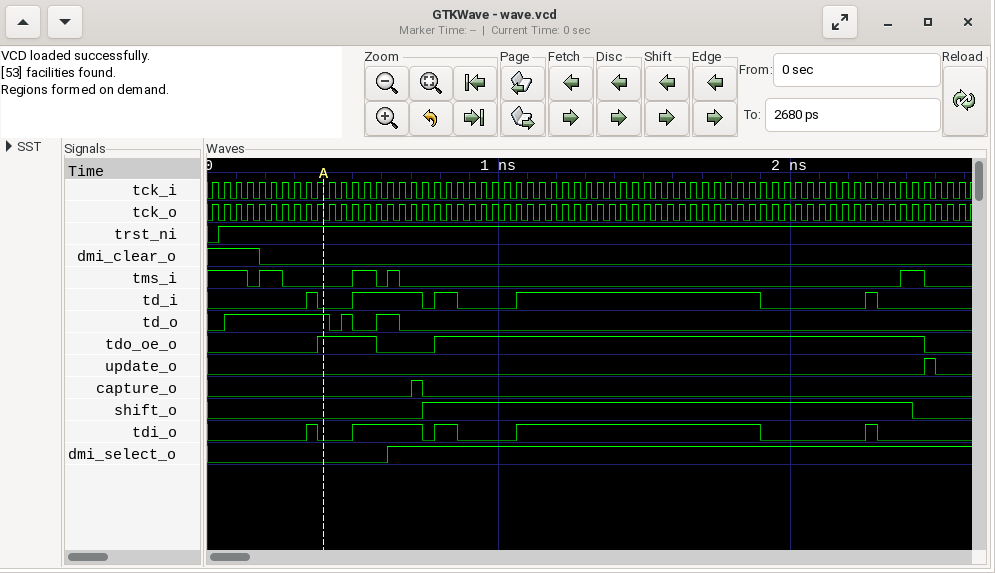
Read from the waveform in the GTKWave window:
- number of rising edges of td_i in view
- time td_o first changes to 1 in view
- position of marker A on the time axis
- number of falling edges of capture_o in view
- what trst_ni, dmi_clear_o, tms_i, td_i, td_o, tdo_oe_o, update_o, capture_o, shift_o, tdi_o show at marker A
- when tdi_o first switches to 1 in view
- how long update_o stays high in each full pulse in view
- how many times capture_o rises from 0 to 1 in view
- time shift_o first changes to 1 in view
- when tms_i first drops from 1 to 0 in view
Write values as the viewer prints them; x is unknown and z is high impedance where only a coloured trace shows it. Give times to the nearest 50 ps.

5
50 ps
400 ps
1
trst_ni=1, dmi_clear_o=0, tms_i=0, td_i=0, td_o=1, tdo_oe_o=1, update_o=0, capture_o=0, shift_o=0, tdi_o=0
350 ps
50 ps
1
750 ps
150 ps
